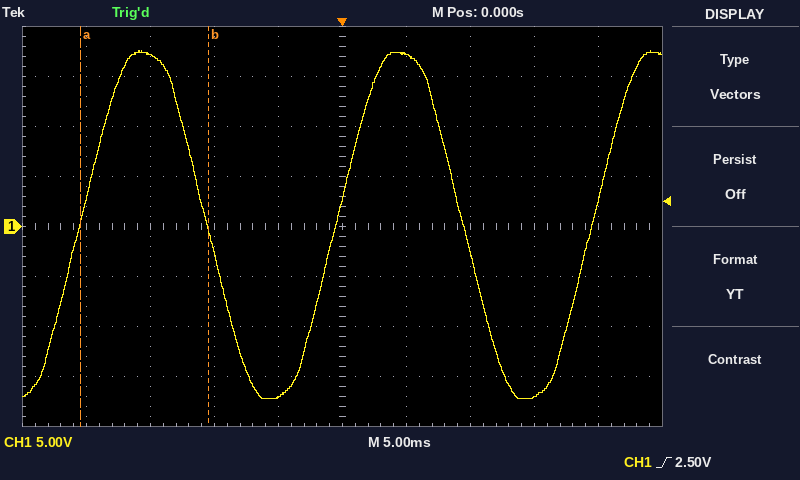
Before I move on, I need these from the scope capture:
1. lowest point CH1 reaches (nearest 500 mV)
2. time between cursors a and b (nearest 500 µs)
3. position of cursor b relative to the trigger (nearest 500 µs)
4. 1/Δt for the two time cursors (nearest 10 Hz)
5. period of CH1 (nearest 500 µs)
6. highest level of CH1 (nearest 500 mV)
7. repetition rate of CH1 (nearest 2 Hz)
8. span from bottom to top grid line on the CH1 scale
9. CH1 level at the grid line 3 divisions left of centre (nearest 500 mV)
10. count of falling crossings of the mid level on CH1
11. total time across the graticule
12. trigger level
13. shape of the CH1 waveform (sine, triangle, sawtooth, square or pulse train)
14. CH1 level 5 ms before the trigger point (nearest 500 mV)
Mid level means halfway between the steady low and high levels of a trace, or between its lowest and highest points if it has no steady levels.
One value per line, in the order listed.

-17.0 V
10.0 ms
-10.5 ms
100 Hz
20.0 ms
17.5 V
50 Hz
40 V
17.0 V
2
50 ms
2.50 V
sine
-17.0 V
